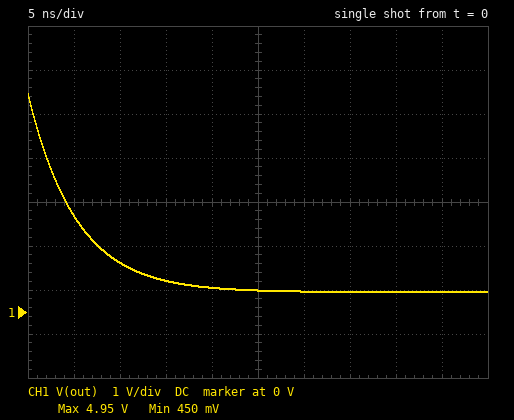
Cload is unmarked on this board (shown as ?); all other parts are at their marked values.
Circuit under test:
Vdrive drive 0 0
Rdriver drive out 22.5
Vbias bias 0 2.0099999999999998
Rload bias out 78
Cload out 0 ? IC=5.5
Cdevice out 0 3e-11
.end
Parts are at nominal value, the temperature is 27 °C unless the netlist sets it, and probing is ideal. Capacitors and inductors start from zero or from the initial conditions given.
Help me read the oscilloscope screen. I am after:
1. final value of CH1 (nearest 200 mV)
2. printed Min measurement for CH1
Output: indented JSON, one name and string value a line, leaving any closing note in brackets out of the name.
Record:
{
  "final value of CH1": "400 mV",
  "printed Min measurement for CH1": "450 mV"
}
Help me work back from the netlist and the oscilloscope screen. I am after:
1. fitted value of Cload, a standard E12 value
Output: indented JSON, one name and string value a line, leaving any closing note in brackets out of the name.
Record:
{
  "fitted value of Cload, a standard E12 value": "270 pF"
}
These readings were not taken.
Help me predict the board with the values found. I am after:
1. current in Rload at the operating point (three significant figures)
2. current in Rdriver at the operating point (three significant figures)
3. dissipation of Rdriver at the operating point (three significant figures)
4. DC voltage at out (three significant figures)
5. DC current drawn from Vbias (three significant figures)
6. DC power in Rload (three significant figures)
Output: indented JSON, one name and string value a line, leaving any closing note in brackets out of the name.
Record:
{
  "current in Rload at the operating point": "20.0 mA",
  "current in Rdriver at the operating point": "20.0 mA",
  "dissipation of Rdriver at the operating point": "9.00 mW",
  "DC voltage at out": "450 mV",
  "DC current drawn from Vbias": "20.0 mA",
  "DC power in Rload": "31.2 mW"
}
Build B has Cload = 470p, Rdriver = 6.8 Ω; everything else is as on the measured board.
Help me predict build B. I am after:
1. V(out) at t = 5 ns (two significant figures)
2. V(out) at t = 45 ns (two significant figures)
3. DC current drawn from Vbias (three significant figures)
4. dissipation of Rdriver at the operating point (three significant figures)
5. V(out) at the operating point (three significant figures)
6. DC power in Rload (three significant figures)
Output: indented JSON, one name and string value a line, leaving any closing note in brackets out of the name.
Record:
{
  "V(out) at t = 5 ns": "1.2 V",
  "V(out) at t = 45 ns": "160 mV",
  "DC current drawn from Vbias": "23.7 mA",
  "dissipation of Rdriver at the operating point": "3.82 mW",
  "V(out) at the operating point": "161 mV",
  "DC power in Rload": "43.8 mW"
}
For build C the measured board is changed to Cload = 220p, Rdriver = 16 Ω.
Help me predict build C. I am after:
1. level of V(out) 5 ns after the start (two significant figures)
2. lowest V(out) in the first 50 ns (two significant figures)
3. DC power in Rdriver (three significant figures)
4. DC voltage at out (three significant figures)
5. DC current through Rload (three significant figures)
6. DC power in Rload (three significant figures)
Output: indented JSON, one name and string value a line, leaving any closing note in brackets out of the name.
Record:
{
  "level of V(out) 5 ns after the start": "1.3 V",
  "lowest V(out) in the first 50 ns": "340 mV",
  "DC power in Rdriver": "7.32 mW",
  "DC voltage at out": "342 mV",
  "DC current through Rload": "21.4 mA",
  "DC power in Rload": "35.7 mW"
}
